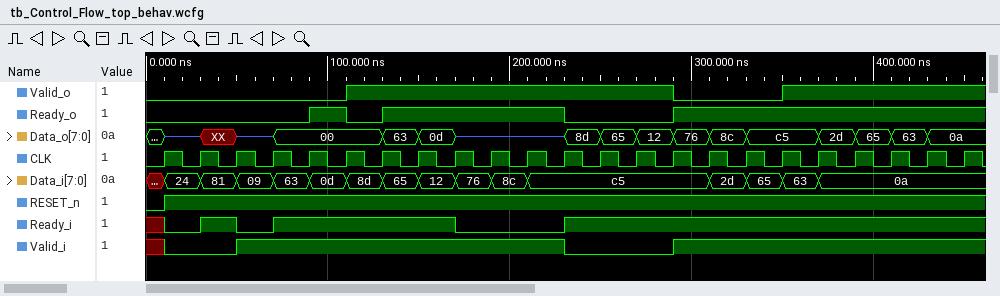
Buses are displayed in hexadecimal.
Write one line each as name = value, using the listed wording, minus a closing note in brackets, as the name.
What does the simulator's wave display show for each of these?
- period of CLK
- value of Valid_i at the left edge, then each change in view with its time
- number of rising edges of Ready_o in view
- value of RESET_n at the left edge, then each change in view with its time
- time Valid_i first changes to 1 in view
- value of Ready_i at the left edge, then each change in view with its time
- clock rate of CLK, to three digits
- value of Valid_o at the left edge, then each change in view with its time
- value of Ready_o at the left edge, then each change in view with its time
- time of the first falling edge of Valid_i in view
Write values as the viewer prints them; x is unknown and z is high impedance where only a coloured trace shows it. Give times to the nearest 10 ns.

period of CLK = 20 ns
value of Valid_i at the left edge, then each change in view with its time = x, 0 at 10 ns, 1 at 50 ns, 0 at 230 ns, 1 at 290 ns
number of rising edges of Ready_o in view = 3
value of RESET_n at the left edge, then each change in view with its time = 0, 1 at 10 ns
time Valid_i first changes to 1 in view = 50 ns
value of Ready_i at the left edge, then each change in view with its time = x, 0 at 10 ns, 1 at 30 ns, 0 at 50 ns, 1 at 70 ns, 0 at 170 ns, 1 at 230 ns
clock rate of CLK, to three digits = 50.0 MHz
value of Valid_o at the left edge, then each change in view with its time = 0, 1 at 110 ns, 0 at 290 ns, 1 at 350 ns
value of Ready_o at the left edge, then each change in view with its time = 0, 1 at 90 ns, 0 at 110 ns, 1 at 130 ns, 0 at 230 ns, 1 at 290 ns
time of the first falling edge of Valid_i in view = 230 ns
